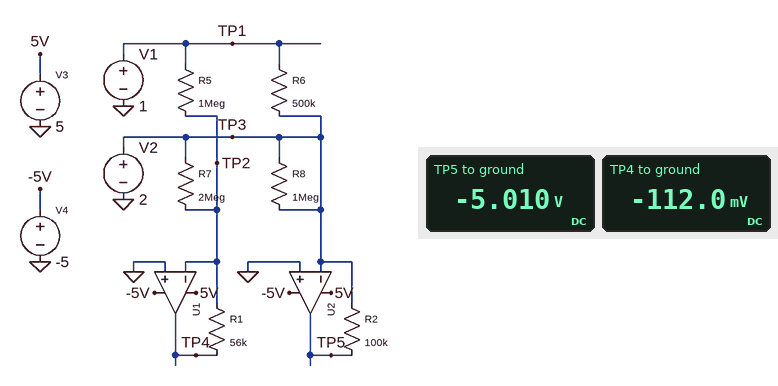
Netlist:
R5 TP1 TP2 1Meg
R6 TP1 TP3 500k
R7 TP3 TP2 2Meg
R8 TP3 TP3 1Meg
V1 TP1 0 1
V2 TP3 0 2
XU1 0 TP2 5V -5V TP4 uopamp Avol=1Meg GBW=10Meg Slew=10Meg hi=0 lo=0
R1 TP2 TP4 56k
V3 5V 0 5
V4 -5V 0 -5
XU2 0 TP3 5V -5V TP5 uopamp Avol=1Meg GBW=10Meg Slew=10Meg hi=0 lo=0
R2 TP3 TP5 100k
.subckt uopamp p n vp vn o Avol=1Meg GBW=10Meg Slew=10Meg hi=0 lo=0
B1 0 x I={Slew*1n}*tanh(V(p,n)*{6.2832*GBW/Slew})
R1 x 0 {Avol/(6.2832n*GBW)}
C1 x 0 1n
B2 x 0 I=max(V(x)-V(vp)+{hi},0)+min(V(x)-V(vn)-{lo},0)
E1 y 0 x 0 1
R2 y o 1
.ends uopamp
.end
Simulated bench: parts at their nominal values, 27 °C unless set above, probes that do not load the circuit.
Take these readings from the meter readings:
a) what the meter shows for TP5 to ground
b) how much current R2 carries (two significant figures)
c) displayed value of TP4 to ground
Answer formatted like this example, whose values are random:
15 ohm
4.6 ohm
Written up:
-5.010 V
70 µA
-112.0 mV
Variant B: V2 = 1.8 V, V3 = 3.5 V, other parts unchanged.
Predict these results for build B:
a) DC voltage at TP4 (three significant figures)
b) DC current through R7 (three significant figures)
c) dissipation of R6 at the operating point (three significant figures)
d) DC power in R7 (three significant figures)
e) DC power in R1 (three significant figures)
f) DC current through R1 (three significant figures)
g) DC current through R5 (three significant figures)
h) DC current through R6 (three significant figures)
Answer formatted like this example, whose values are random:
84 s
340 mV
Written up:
-106 mV
900 nA
1.28 µW
1.62 µW
202 nW
1.90 µA
1.00 µA
1.60 µA
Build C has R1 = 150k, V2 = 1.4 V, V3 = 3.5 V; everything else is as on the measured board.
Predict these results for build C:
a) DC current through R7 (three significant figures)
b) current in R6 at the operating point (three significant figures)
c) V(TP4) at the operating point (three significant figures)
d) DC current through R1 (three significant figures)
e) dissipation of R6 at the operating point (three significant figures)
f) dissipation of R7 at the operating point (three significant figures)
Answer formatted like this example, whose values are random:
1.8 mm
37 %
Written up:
700 nA
800 nA
-255 mV
1.70 µA
320 nW
980 nW
